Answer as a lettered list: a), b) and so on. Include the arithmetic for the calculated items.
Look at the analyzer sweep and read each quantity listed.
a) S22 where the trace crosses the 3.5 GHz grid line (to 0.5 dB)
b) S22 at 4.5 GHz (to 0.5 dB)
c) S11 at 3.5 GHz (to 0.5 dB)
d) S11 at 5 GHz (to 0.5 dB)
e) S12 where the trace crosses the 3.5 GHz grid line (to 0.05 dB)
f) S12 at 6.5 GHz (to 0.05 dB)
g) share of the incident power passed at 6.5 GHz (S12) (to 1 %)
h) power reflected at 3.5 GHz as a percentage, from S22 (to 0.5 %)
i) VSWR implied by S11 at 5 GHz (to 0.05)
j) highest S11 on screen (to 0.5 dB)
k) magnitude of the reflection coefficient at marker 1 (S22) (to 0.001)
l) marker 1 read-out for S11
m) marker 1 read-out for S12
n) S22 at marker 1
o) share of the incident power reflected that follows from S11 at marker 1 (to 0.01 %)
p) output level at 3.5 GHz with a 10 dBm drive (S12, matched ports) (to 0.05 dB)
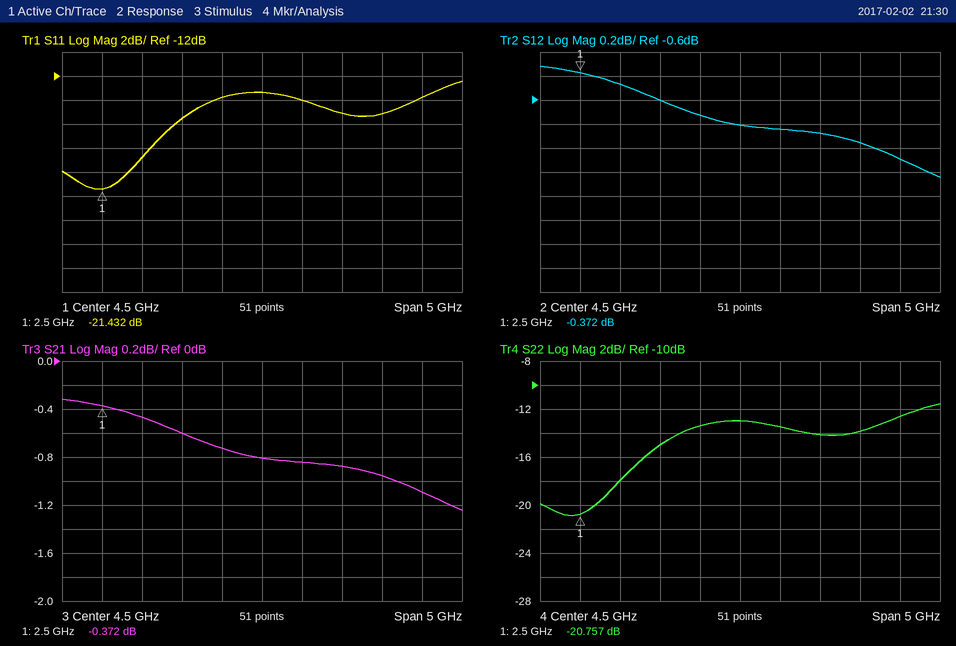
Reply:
a) -15.0 dB
b) -13.0 dB
c) -15.5 dB
d) -14.0 dB
e) -0.60 dB
f) -1.10 dB
g) 10^(-1.1/10) ≈ 78 %
h) 10^(-15/10) ≈ 3.16 %, so 3.0 % to the nearest 0.5 %
i) |Γ| = 10^(-14/20) = 0.1995; VSWR = (1 + 0.1995)/(1 − 0.1995) ≈ 1.50
j) -12.5 dB
k) 10^(-20.757/20) ≈ 0.092
l) -21.432 dB
m) -0.372 dB
n) -20.757 dB
o) 10^(-21.432/10) ≈ 0.72 %
p) 10 dBm + (-0.60 dB) = 9.40 dBm
